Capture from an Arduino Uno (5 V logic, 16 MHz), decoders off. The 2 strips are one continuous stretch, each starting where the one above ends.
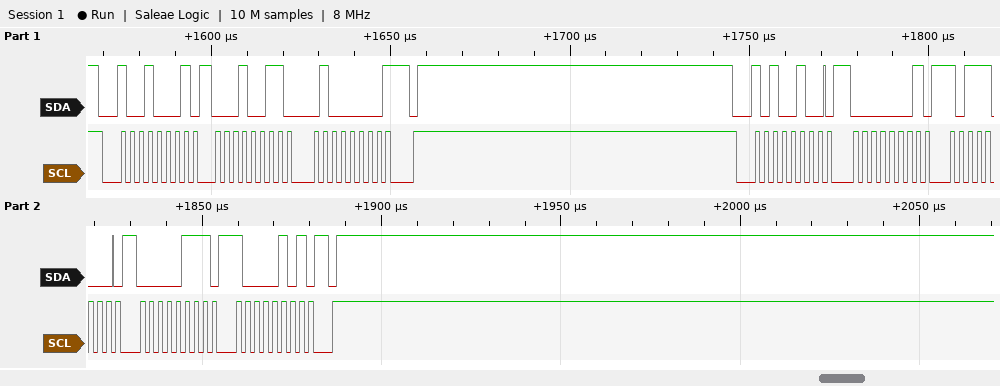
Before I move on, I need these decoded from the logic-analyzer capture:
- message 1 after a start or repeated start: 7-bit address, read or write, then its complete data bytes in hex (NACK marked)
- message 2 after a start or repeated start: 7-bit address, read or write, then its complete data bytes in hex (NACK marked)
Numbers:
0x48 read: 13 40 NACK
0x52 write: 01 B8 07 85
